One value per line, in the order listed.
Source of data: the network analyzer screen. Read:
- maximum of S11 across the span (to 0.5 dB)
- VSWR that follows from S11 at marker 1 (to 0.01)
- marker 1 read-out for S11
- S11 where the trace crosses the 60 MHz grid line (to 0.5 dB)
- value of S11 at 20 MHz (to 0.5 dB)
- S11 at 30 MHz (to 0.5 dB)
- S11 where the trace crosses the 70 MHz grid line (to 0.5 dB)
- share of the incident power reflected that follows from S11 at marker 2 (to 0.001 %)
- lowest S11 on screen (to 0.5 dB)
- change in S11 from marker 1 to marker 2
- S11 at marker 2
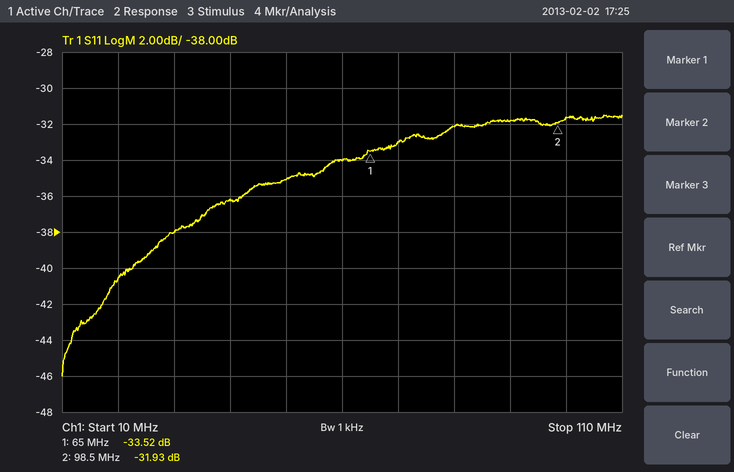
-31.5 dB
1.04
-33.52 dB
-34.0 dB
-40.5 dB
-38.0 dB
-33.0 dB
0.064 %
-46.0 dB
1.59 dB
-31.93 dB
